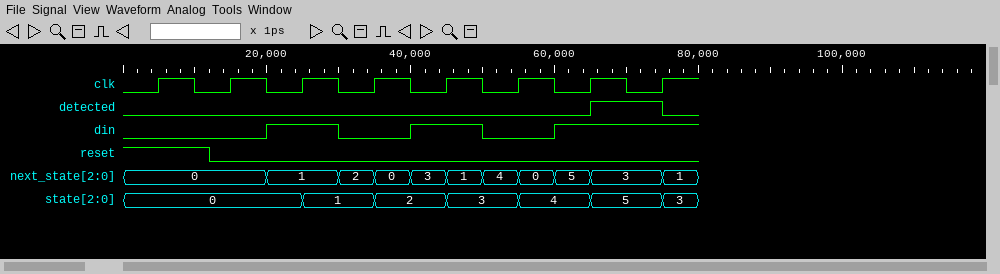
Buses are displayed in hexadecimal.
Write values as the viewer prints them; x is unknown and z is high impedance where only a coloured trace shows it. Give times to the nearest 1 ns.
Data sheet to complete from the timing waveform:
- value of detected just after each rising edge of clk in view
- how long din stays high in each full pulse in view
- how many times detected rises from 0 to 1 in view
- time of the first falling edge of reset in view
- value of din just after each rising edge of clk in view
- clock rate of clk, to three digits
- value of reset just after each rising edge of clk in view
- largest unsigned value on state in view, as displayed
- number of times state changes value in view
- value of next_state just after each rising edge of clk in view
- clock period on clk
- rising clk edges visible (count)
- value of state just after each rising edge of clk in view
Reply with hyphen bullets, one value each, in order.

- 0 0 0 0 0 0 1 0
- 10 ns, 10 ns
- 1
- 12 ns
- 0 0 1 0 1 0 1 1
- 100 MHz
- 1 0 0 0 0 0 0 0
- 5
- 6
- 0, 0, 1, 0, 1, 0, 3, 1
- 10 ns
- 8
- 0, 0, 1, 2, 3, 4, 5, 3
